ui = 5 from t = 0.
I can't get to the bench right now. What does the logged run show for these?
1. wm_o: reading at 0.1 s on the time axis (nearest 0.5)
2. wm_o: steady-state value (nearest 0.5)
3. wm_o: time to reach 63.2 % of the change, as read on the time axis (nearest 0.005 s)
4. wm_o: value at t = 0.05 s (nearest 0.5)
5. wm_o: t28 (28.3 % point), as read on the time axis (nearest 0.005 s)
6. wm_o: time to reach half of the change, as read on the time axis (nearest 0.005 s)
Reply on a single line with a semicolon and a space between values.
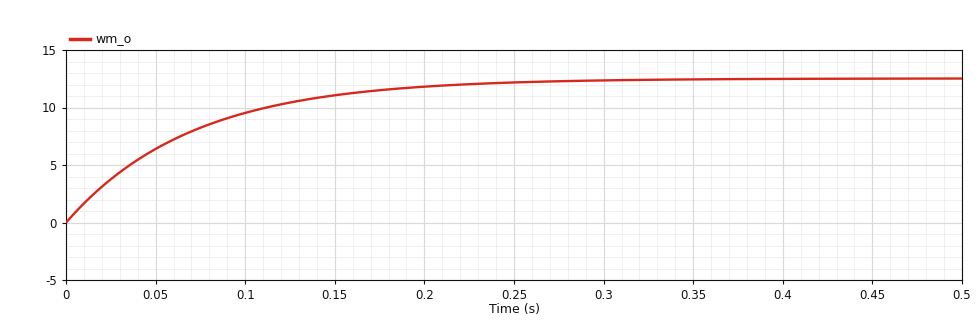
9.5; 12.5; 0.070 s; 6.5; 0.025 s; 0.050 s
